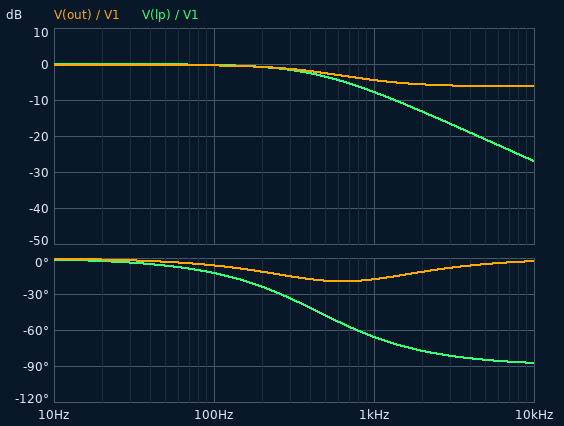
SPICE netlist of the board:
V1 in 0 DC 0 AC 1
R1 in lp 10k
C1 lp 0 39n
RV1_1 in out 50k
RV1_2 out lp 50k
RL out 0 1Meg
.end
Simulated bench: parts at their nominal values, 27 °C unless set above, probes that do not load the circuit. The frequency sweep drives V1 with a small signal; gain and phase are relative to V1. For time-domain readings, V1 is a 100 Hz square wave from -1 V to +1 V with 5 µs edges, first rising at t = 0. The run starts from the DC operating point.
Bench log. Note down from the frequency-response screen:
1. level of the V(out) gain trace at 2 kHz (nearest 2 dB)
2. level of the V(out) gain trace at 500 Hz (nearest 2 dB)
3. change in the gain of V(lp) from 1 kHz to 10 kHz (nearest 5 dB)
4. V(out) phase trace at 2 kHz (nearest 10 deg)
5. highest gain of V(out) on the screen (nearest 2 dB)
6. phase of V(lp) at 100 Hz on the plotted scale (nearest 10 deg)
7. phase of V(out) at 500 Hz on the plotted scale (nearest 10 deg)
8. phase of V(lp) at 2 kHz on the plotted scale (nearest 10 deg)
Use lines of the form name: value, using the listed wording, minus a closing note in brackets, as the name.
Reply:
level of the V(out) gain trace at 2 kHz: -6 dB
level of the V(out) gain trace at 500 Hz: -2 dB
change in the gain of V(lp) from 1 kHz to 10 kHz: -20 dB
V(out) phase trace at 2 kHz: -10 deg
highest gain of V(out) on the screen: 0 dB
phase of V(lp) at 100 Hz on the plotted scale: -10 deg
phase of V(out) at 500 Hz on the plotted scale: -20 deg
phase of V(lp) at 2 kHz on the plotted scale: -80 deg
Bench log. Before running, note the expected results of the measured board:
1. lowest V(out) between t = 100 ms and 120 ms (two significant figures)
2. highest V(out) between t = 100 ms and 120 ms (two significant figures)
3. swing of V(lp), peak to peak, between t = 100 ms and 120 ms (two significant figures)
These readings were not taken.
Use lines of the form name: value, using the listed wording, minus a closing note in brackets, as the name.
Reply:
lowest V(out) between t = 100 ms and 120 ms: -970 mV
highest V(out) between t = 100 ms and 120 ms: 970 mV
swing of V(lp), peak to peak, between t = 100 ms and 120 ms: 2.0 V
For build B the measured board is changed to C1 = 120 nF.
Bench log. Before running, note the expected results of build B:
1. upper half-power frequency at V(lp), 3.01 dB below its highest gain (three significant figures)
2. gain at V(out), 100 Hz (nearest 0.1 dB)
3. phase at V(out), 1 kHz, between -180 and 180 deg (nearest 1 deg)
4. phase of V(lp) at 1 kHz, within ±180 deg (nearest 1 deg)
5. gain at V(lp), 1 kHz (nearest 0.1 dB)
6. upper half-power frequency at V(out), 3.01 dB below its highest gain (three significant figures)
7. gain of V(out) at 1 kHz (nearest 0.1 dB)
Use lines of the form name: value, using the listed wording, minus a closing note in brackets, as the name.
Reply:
upper half-power frequency at V(lp), 3.01 dB below its highest gain: 146 Hz
gain at V(out), 100 Hz: -1.4 dB
phase at V(out), 1 kHz, between -180 and 180 deg: -8 deg
phase of V(lp) at 1 kHz, within ±180 deg: -82 deg
gain at V(lp), 1 kHz: -16.8 dB
upper half-power frequency at V(out), 3.01 dB below its highest gain: 207 Hz
gain of V(out) at 1 kHz: -6.0 dB
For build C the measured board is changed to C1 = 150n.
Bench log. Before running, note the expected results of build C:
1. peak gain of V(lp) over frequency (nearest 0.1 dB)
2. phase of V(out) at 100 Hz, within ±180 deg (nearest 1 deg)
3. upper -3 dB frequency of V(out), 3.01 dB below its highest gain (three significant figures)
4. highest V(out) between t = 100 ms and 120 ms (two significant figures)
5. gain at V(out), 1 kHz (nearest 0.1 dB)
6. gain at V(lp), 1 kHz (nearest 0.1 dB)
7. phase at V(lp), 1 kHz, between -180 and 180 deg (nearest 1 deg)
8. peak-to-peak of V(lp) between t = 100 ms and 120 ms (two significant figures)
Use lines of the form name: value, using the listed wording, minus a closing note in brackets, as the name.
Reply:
peak gain of V(lp) over frequency: 0 dB
phase of V(out) at 100 Hz, within ±180 deg: -17 deg
upper -3 dB frequency of V(out), 3.01 dB below its highest gain: 166 Hz
highest V(out) between t = 100 ms and 120 ms: 950 mV
gain at V(out), 1 kHz: -6.1 dB
gain at V(lp), 1 kHz: -18.7 dB
phase at V(lp), 1 kHz, between -180 and 180 deg: -83 deg
peak-to-peak of V(lp) between t = 100 ms and 120 ms: 1.9 V
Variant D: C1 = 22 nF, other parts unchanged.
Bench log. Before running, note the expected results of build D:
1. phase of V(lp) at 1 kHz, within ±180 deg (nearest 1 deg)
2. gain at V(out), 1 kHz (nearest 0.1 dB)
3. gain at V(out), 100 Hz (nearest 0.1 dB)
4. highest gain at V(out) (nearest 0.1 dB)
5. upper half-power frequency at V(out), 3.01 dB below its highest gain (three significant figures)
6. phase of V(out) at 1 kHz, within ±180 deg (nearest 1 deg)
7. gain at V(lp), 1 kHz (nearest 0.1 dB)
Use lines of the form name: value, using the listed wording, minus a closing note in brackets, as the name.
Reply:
phase of V(lp) at 1 kHz, within ±180 deg: -51 deg
gain at V(out), 1 kHz: -2.9 dB
gain at V(out), 100 Hz: -0.3 dB
highest gain at V(out): -0.2 dB
upper half-power frequency at V(out), 3.01 dB below its highest gain: 1.13 kHz
phase of V(out) at 1 kHz, within ±180 deg: -19 deg
gain at V(lp), 1 kHz: -4.1 dB
